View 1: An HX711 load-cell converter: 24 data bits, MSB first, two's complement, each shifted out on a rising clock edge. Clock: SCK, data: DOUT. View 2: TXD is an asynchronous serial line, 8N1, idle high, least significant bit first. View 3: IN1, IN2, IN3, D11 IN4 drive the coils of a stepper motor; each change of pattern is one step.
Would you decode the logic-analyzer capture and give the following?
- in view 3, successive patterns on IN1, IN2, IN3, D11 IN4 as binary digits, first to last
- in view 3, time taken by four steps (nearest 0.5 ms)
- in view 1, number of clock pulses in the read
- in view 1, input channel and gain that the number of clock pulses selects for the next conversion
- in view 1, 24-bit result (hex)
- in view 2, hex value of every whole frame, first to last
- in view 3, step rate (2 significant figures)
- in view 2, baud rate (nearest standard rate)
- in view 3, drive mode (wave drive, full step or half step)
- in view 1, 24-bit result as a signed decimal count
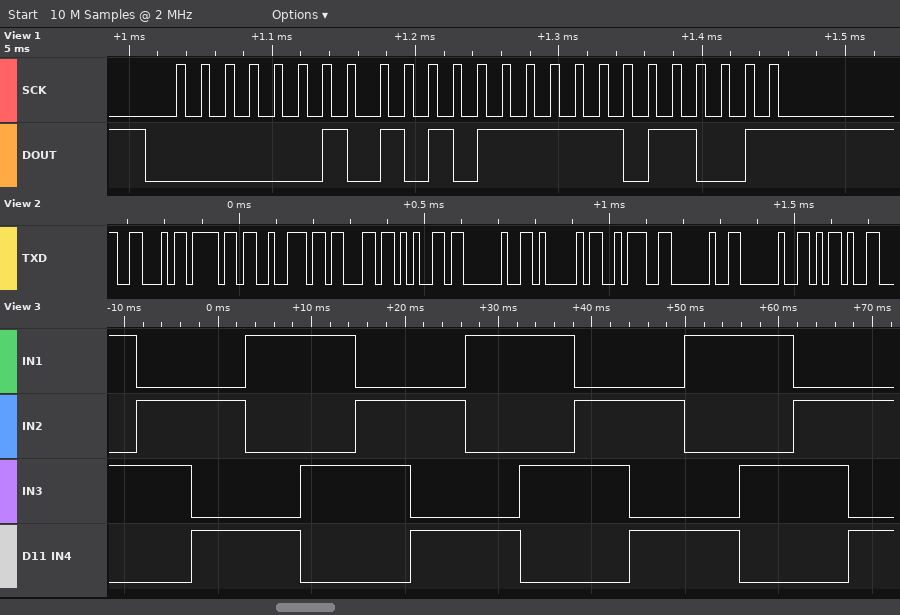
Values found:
1010 0110 0101 1001 1010 0110 0101 1001 1010 0110 0101 1001 1010 0110 0101
23.5 ms
25
channel A, gain 128
0x02AFD9
0x46 0x6F 0x72 0x63 0x65 0x20 0x41 0x3A 0x20 0x20 0x2D
170 steps/s
57600 baud
full step
176089
